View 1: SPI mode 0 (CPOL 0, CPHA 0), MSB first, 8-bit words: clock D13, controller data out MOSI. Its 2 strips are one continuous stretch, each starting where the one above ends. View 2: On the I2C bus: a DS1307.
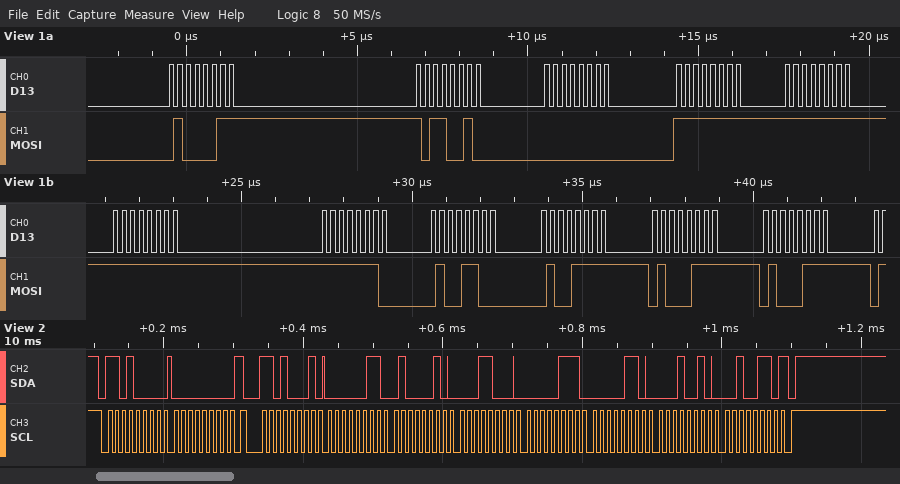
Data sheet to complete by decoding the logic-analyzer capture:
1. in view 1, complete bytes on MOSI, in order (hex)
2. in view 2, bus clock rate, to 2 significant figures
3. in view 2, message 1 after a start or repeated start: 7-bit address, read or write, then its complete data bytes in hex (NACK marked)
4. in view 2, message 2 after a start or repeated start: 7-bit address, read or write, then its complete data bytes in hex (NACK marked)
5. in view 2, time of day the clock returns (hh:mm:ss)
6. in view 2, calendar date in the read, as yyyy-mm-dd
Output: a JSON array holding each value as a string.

["43 B2 00 FF FF FF FE 4C 4F 47 47", "100 kHz", "0x68 write: 00", "0x68 read: 03 42 18 07 06 12 26 NACK", "18:42:03", "2026-12-06"]
